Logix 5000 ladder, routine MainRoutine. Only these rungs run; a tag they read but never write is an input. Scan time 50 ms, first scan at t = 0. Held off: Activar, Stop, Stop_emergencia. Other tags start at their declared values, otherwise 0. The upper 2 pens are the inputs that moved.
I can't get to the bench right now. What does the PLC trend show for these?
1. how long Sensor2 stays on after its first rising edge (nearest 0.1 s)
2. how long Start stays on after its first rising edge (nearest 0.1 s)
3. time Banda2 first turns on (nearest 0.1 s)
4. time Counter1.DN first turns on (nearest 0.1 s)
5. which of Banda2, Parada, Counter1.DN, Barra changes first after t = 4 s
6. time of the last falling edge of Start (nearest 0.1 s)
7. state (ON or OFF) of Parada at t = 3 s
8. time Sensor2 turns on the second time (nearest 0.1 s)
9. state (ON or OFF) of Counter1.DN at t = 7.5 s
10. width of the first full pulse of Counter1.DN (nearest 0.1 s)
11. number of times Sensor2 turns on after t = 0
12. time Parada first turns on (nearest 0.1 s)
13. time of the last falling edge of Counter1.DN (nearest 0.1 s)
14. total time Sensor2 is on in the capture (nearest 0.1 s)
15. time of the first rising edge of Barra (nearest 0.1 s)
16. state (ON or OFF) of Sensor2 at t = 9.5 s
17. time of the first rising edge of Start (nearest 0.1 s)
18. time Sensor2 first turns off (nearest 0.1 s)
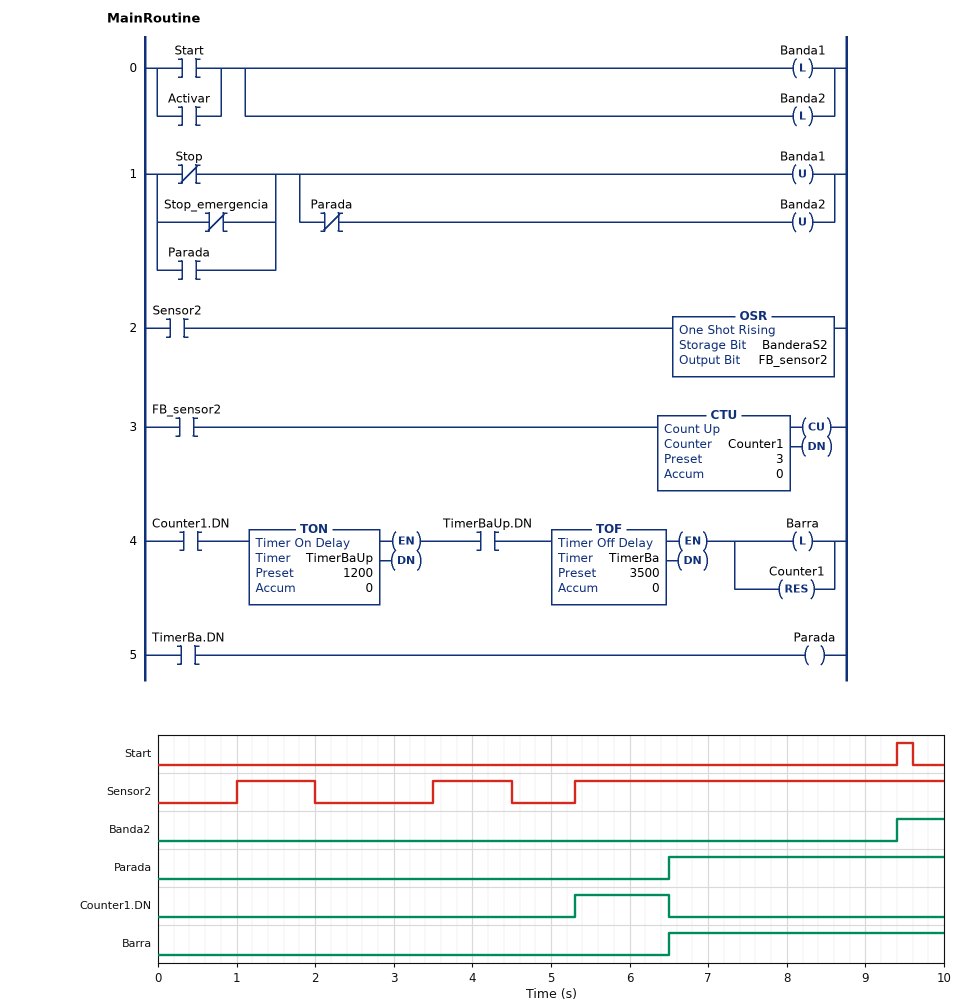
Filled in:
1.0 s
0.2 s
9.4 s
5.3 s
Counter1.DN
9.6 s
OFF
3.5 s
OFF
1.2 s
3
6.5 s
6.5 s
6.7 s
6.5 s
ON
9.4 s
2.0 s
